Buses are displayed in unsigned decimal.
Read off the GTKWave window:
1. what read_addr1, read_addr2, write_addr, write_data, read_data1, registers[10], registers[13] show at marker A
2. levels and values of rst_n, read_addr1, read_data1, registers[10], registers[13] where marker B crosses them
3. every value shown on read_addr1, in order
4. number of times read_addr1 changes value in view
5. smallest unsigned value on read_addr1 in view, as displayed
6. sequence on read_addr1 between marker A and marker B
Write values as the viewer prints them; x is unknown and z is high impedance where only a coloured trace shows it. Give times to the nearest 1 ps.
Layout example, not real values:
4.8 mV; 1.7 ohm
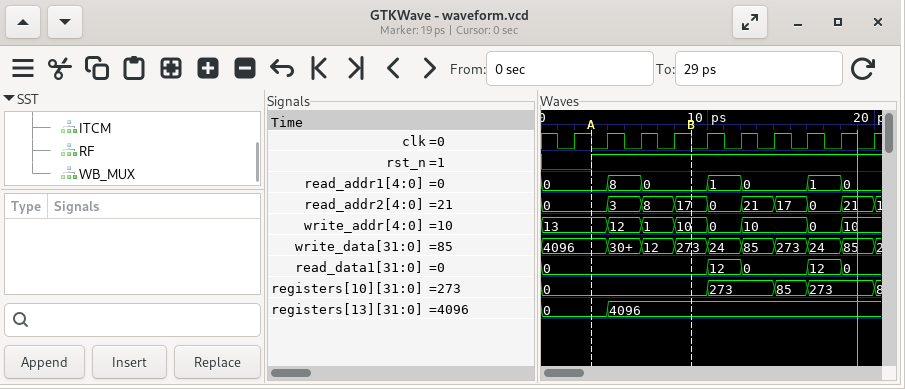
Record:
read_addr1=0, read_addr2=0, write_addr=13, write_data=4096, read_data1=0, registers[10]=0, registers[13]=0; rst_n=1, read_addr1=0, read_data1=0, registers[10]=0, registers[13]=4096; 0, 8, 0, 1, 0, 1, 0; 6; 0; 0, 8, 0
